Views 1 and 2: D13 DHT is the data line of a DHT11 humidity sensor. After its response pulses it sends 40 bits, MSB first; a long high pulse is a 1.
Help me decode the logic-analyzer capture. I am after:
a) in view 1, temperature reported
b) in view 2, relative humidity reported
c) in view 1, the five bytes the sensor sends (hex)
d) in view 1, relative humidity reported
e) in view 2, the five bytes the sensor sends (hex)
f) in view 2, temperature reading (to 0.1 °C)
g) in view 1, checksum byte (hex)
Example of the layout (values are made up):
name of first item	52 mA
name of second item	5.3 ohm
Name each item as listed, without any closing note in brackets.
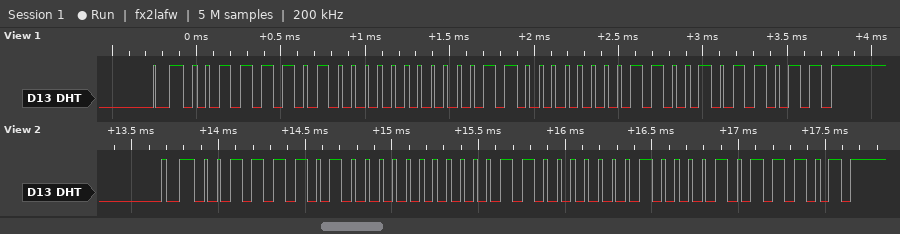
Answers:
in view 1, temperature reported	24.6 °C
in view 2, relative humidity reported	61 %
in view 1, the five bytes the sensor sends	3D 00 18 06 5B
in view 1, relative humidity reported	61 %
in view 2, the five bytes the sensor sends	3D 00 18 08 5D
in view 2, temperature reading	24.8 °C
in view 1, checksum byte	0x5B
